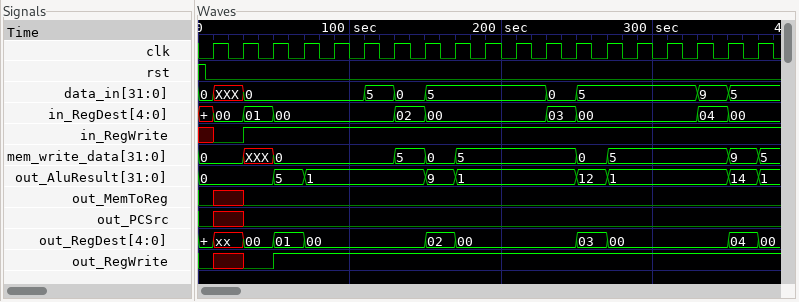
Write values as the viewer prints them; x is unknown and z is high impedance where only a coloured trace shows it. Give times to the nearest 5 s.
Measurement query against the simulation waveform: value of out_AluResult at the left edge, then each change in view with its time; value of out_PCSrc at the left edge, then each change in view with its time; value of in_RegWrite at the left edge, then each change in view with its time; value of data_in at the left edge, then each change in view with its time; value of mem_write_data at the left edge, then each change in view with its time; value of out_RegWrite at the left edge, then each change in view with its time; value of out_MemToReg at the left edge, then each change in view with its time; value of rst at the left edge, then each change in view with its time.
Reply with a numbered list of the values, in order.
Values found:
1. 0, 5 at 50 s, 1 at 70 s, 9 at 150 s, 1 at 170 s, 12 at 250 s, 1 at 270 s, 14 at 350 s, 1 at 370 s
2. 0, x at 10 s, 0 at 30 s
3. x, 0 at 10 s, 1 at 30 s
4. 0, XXX at 10 s, 0 at 30 s, 5 at 110 s, 0 at 130 s, 5 at 150 s, 0 at 230 s, 5 at 250 s, 9 at 330 s, 5 at 350 s
5. 0, XXX at 30 s, 0 at 50 s, 5 at 130 s, 0 at 150 s, 5 at 170 s, 0 at 250 s, 5 at 270 s, 9 at 350 s, 5 at 370 s
6. 0, x at 10 s, 0 at 30 s, 1 at 50 s
7. 0, x at 10 s, 0 at 30 s
8. 1, 0 at 5 s
